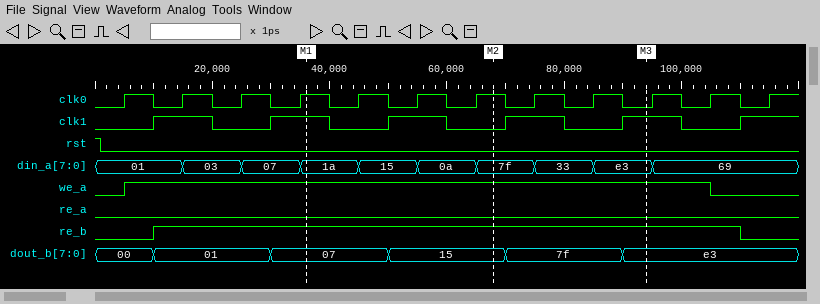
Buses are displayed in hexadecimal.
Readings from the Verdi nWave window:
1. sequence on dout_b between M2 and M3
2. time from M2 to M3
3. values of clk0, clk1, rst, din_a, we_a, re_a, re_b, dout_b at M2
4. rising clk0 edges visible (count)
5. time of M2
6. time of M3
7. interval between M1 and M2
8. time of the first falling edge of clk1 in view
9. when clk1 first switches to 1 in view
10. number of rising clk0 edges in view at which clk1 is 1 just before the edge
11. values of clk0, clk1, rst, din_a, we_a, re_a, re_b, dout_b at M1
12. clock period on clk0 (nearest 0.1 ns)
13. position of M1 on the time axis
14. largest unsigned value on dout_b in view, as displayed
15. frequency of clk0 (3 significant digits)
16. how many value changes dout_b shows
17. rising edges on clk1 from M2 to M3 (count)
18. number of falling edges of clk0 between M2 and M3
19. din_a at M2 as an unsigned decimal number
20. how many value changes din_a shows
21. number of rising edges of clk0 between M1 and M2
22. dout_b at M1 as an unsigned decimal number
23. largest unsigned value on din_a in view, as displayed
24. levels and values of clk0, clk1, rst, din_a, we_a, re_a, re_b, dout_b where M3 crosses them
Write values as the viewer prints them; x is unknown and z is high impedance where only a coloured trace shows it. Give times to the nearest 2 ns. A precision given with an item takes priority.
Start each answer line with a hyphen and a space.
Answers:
- 15, 7f, e3
- 26 ns
- clk0=1, clk1=0, rst=0, din_a=7f, we_a=1, re_a=0, re_b=1, dout_b=15
- 12
- 68 ns
- 94 ns
- 32 ns
- 20 ns
- 10 ns
- 6
- clk0=1, clk1=1, rst=0, din_a=1a, we_a=1, re_a=0, re_b=1, dout_b=07
- 10 ns
- 36 ns
- e3
- 100 MHz
- 5
- 2
- 3
- 127
- 9
- 3
- 7
- e3
- clk0=0, clk1=1, rst=0, din_a=e3, we_a=1, re_a=0, re_b=1, dout_b=e3
